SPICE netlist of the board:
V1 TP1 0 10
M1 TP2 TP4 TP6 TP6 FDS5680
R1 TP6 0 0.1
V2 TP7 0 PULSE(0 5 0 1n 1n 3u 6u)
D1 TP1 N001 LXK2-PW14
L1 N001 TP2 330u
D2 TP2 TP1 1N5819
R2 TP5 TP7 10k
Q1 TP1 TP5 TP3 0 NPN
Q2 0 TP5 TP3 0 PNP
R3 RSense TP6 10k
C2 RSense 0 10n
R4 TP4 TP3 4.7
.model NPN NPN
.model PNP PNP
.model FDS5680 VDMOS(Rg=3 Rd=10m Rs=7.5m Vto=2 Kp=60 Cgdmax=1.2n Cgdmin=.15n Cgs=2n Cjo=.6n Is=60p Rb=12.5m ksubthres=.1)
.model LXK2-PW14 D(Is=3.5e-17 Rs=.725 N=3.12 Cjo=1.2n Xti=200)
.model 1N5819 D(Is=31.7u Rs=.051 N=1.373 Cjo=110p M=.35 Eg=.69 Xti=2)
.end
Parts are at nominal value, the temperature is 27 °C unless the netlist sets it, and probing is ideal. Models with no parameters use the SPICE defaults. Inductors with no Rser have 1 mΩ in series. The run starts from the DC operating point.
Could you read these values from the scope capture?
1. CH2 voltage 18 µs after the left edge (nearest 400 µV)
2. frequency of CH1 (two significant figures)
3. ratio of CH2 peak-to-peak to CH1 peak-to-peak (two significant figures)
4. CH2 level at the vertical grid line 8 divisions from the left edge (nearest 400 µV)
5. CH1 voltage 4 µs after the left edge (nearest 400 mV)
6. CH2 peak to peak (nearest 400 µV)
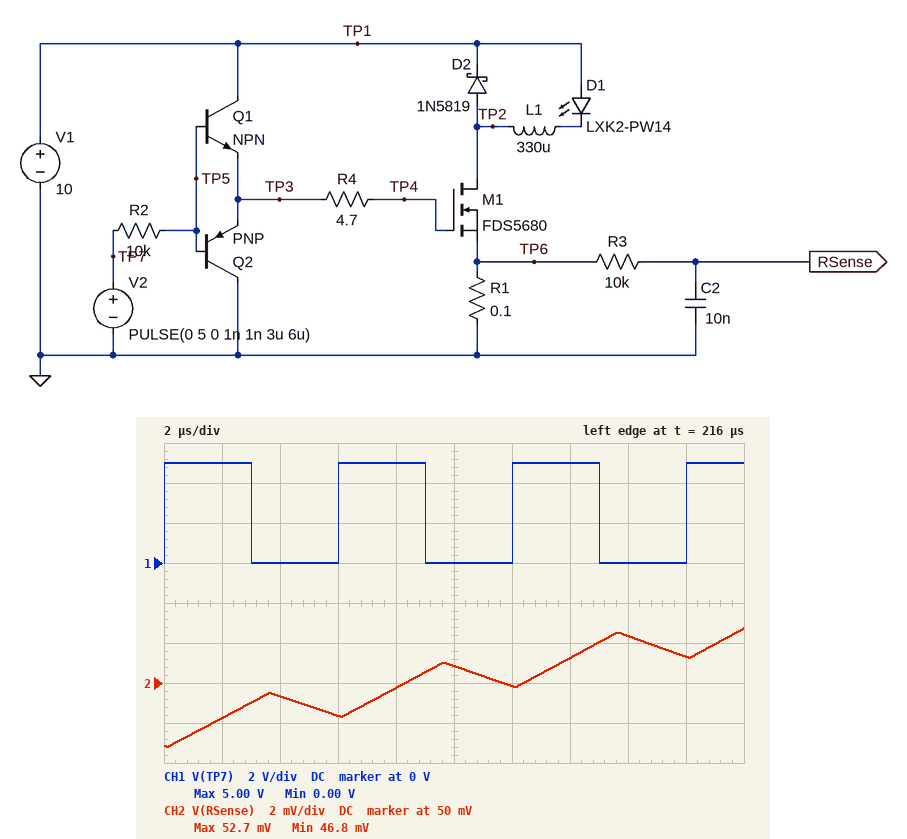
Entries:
51.2 mV
170 kHz
0.0012
52.4 mV
0 V
6.0 mV
